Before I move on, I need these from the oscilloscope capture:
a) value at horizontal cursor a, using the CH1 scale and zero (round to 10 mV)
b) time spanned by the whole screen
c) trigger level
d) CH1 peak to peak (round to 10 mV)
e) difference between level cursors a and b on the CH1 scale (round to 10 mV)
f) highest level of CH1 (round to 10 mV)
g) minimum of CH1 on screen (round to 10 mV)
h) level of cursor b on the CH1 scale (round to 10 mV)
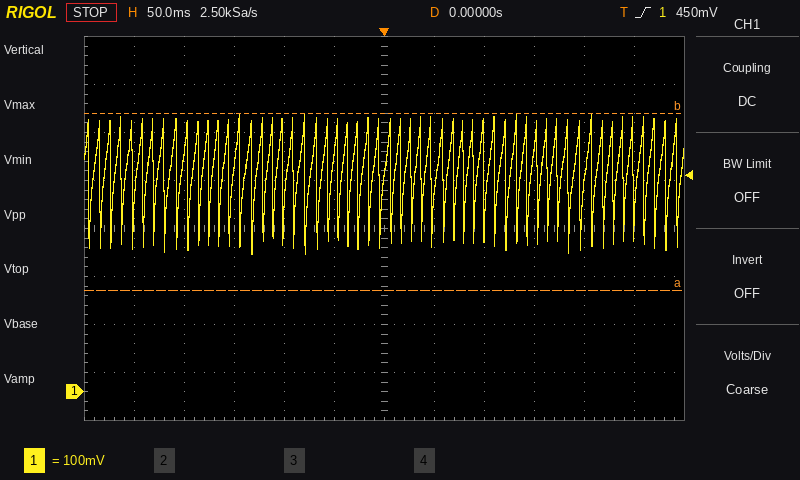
210 mV
600 ms
450 mV
290 mV
370 mV
580 mV
290 mV
580 mV
